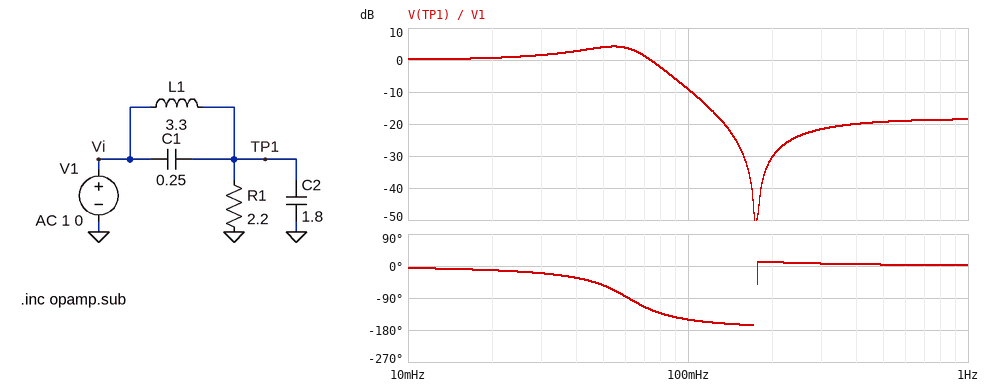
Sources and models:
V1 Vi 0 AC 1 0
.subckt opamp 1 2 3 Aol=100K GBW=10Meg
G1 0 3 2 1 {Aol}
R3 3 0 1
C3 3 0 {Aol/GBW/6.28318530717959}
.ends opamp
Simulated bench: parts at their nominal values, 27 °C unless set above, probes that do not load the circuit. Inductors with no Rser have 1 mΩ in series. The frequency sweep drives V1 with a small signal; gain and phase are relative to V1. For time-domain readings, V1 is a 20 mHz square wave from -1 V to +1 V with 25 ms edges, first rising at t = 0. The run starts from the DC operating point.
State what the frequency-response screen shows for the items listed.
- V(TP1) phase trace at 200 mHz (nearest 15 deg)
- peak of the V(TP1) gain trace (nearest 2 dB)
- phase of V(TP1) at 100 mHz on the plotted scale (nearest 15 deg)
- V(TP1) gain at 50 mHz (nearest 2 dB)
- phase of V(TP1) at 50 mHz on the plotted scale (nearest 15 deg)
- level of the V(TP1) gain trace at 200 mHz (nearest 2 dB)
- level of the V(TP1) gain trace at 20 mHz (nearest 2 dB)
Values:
15 deg
4 dB
-150 deg
4 dB
-60 deg
-30 dB
0 dB
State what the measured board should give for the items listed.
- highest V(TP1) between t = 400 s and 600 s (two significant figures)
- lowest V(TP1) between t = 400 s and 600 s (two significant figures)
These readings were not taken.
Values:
1.7 V
-1.7 V
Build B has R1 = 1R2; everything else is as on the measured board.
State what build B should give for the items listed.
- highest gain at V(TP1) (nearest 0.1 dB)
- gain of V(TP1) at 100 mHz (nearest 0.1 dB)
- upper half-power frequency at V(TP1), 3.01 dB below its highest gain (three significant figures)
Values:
0.5 dB
-11.0 dB
65.7 mHz
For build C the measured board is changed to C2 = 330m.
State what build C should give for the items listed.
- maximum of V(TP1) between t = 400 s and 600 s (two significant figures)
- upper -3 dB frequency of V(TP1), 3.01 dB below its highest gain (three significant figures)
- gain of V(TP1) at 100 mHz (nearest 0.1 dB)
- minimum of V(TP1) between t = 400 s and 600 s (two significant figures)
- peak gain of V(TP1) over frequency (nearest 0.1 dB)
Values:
1.2 V
98.6 mHz
-3.2 dB
-1.2 V
0 dB
